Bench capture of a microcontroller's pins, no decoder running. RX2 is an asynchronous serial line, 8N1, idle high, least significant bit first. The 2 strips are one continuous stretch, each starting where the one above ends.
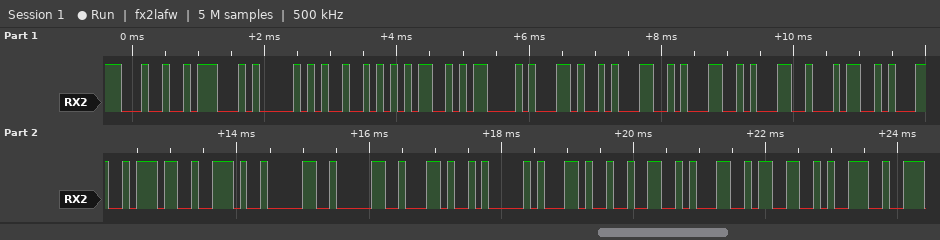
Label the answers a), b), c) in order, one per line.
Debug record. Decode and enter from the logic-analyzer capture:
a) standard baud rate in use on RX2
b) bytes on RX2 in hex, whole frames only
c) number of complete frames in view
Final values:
a) 9600 baud
b) 24 47 50 52 4D 43 2C 31 31 31 34 31 37 2E 30 30 2C 41 2C 32 31 33 39
c) 23
